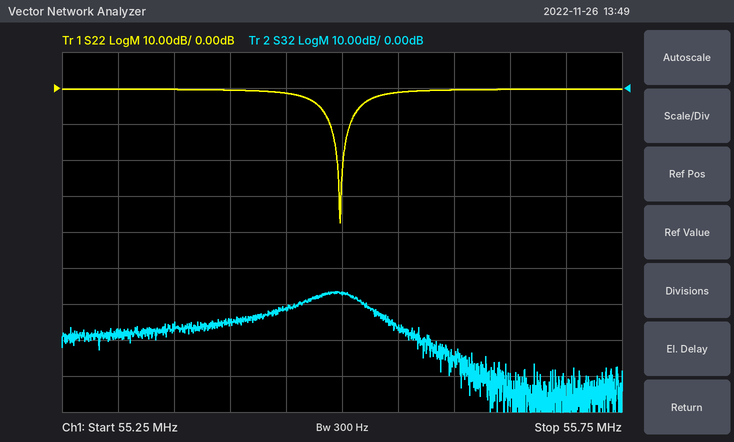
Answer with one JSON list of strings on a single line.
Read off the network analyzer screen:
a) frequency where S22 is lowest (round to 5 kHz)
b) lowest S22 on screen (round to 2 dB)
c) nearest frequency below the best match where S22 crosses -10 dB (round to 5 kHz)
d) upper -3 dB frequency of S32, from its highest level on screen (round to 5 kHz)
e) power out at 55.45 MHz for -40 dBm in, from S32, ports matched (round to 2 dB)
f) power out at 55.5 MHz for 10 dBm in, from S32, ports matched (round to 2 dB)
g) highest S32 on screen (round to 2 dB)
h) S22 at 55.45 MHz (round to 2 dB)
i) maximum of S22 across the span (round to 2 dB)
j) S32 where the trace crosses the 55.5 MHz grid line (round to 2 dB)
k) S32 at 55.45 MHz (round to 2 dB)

["55.500 MHz", "-38 dB", "55.490 MHz", "55.515 MHz", "-102 dBm", "-48 dBm", "-56 dB", "-2 dB", "0 dB", "-58 dB", "-62 dB"]
